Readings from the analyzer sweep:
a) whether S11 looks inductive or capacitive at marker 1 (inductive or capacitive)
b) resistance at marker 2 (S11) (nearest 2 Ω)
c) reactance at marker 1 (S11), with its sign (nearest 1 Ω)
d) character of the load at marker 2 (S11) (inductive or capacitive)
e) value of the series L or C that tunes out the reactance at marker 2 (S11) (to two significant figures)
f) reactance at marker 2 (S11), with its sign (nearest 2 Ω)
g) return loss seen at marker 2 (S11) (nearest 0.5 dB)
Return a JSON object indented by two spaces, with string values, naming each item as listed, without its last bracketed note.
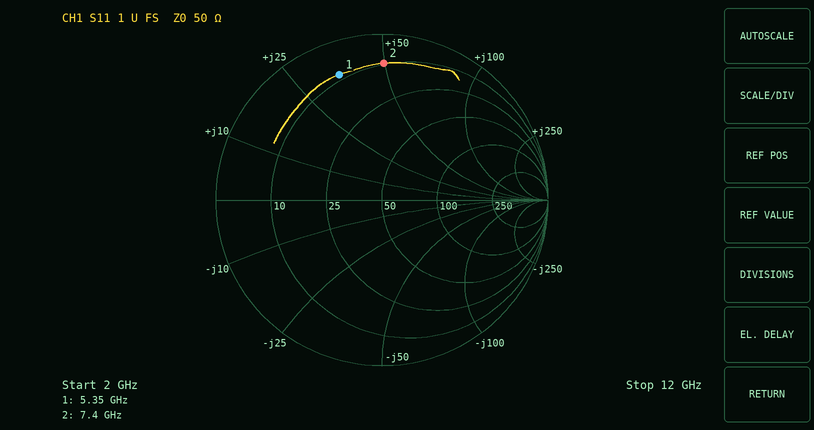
{
  "whether S11 looks inductive or capacitive at marker 1": "inductive",
  "resistance at marker 2 (S11)": "10 Ω",
  "reactance at marker 1 (S11), with its sign": "+35 Ω",
  "character of the load at marker 2 (S11)": "inductive",
  "value of the series L or C that tunes out the reactance at marker 2 (S11)": "430 fF",
  "reactance at marker 2 (S11), with its sign": "+50 Ω",
  "return loss seen at marker 2 (S11)": "1.5 dB"
}
